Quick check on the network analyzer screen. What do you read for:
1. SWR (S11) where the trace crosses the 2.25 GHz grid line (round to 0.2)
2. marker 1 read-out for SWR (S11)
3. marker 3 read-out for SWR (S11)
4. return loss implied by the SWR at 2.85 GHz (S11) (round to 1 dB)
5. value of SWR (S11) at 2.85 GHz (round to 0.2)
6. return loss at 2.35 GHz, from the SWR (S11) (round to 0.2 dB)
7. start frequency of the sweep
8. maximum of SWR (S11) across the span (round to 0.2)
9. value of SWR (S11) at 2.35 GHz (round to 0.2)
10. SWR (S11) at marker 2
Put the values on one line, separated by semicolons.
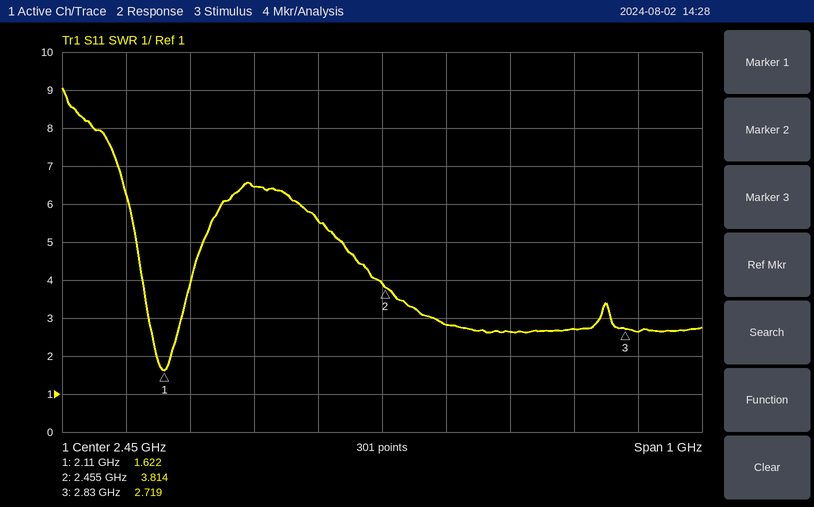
6.4; 1.622; 2.719; 7 dB; 2.6; 3.2 dB; 1.95 GHz; 9.0; 5.6; 3.814
